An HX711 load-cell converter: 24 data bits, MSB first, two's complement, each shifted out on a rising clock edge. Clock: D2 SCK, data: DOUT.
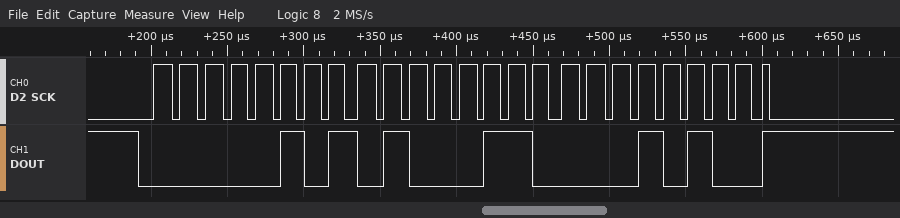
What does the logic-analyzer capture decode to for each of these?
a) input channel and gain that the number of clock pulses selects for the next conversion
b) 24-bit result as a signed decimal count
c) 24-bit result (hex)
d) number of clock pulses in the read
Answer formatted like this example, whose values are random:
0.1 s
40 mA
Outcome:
channel A, gain 128
345620
0x054614
25
